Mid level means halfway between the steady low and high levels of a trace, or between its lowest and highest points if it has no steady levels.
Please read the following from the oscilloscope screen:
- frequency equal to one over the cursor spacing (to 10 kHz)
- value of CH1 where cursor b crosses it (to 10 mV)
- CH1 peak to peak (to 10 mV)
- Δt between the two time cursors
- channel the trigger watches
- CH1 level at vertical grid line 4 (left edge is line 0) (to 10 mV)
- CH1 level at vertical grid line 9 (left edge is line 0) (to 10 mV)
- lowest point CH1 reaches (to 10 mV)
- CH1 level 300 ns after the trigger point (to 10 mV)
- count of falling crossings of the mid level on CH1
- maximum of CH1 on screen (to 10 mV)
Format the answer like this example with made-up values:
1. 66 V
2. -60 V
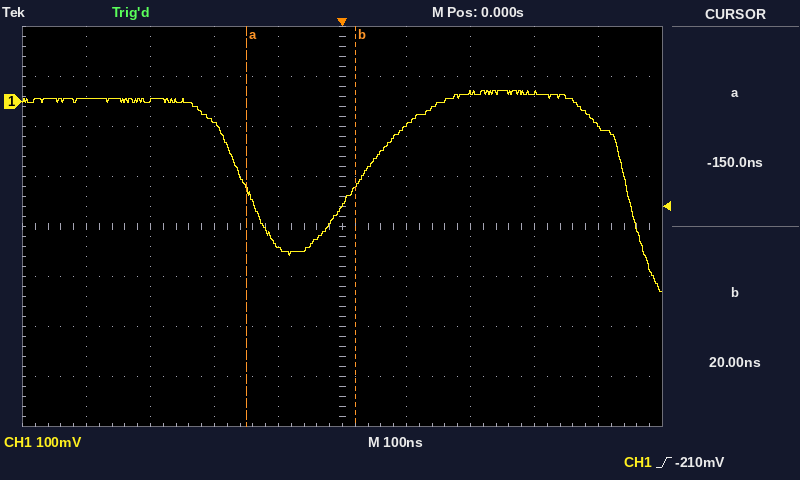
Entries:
1. 5.88 MHz
2. -170 mV
3. 400 mV
4. 170 ns
5. CH1
6. -290 mV
7. -50 mV
8. -380 mV
9. 20 mV
10. 2
11. 20 mV
